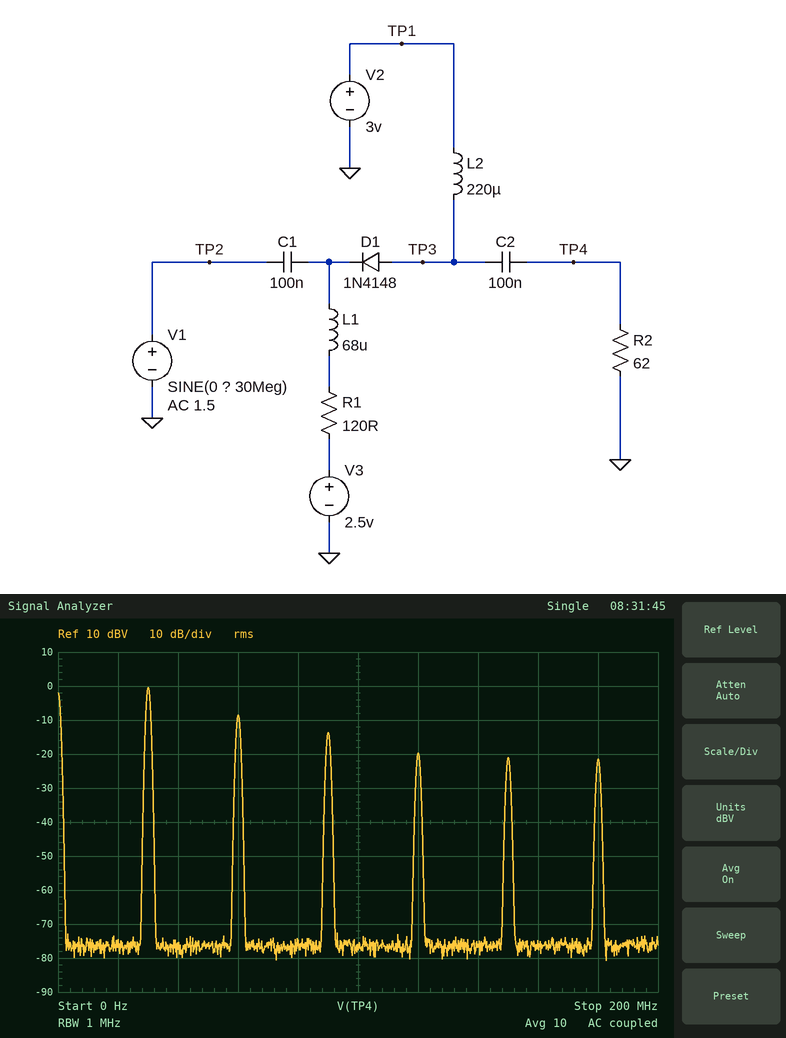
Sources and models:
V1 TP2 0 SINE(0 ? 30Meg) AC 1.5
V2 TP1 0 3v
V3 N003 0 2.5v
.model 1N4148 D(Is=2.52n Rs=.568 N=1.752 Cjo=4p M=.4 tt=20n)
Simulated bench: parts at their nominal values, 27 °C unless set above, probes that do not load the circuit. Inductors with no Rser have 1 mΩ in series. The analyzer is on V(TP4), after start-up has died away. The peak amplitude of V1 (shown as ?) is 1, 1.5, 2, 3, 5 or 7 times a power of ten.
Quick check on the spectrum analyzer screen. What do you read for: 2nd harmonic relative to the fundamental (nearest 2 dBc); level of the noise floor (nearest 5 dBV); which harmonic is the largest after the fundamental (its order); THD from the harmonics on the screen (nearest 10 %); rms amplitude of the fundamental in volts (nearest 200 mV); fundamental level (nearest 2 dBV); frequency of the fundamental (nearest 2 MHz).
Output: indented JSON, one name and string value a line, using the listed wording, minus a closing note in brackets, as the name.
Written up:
{
  "2nd harmonic relative to the fundamental": "-8 dBc",
  "level of the noise floor": "-75 dBV",
  "which harmonic is the largest after the fundamental": "2",
  "THD from the harmonics on the screen": "50 %",
  "rms amplitude of the fundamental in volts": "1.0 V",
  "fundamental level": "0 dBV",
  "frequency of the fundamental": "30 MHz"
}
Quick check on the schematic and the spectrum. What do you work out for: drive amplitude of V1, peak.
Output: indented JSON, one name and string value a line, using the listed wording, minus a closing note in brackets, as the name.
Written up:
{
  "drive amplitude of V1, peak": "2 V"
}
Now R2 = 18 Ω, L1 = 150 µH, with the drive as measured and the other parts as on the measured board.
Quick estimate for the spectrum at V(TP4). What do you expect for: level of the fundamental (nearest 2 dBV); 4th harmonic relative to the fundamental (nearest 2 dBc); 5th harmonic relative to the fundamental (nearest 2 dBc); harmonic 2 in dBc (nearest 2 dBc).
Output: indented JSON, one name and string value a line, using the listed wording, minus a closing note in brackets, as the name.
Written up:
{
  "level of the fundamental": "-6 dBV",
  "4th harmonic relative to the fundamental": "-12 dBc",
  "5th harmonic relative to the fundamental": "-16 dBc",
  "harmonic 2 in dBc": "-2 dBc"
}
